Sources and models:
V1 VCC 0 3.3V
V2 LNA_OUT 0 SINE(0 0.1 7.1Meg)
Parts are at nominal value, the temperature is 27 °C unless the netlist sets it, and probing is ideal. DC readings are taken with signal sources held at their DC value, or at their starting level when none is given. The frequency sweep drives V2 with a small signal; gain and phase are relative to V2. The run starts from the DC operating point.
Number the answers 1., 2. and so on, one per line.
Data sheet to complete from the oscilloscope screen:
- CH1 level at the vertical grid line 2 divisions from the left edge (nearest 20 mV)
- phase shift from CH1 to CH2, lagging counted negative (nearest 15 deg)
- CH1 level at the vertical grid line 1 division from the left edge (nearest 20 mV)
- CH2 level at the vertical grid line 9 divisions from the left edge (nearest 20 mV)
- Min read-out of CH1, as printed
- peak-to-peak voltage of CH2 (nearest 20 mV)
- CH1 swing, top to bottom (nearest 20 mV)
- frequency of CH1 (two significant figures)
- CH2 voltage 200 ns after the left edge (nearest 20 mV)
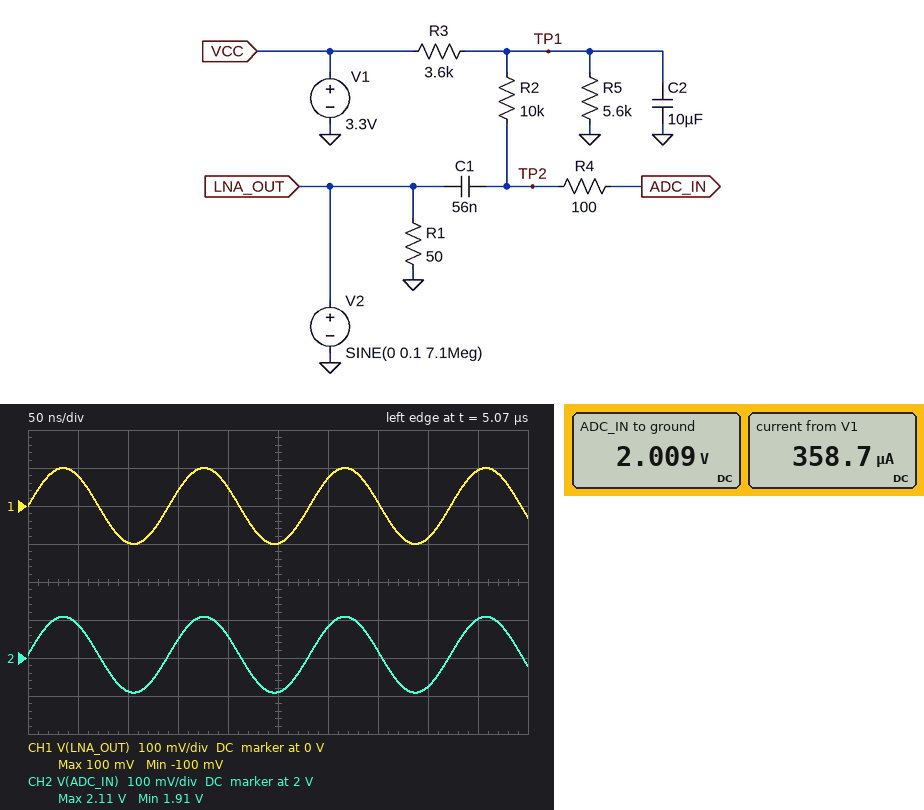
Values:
1. -100 mV
2. 0 deg
3. 80 mV
4. 2.10 V
5. -100 mV
6. 200 mV
7. 200 mV
8. 7.1 MHz
9. 2.06 V
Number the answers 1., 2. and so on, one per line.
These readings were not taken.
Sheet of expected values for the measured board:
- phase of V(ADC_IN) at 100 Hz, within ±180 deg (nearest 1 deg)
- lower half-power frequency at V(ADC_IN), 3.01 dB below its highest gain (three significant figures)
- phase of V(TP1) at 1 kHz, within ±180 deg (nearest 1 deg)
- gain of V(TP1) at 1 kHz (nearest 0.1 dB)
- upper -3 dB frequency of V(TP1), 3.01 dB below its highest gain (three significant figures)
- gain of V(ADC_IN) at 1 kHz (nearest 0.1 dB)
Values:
1. 70 deg
2. 286 Hz
3. -74 deg
4. -56.3 dB
5. 300 Hz
6. -0.3 dB
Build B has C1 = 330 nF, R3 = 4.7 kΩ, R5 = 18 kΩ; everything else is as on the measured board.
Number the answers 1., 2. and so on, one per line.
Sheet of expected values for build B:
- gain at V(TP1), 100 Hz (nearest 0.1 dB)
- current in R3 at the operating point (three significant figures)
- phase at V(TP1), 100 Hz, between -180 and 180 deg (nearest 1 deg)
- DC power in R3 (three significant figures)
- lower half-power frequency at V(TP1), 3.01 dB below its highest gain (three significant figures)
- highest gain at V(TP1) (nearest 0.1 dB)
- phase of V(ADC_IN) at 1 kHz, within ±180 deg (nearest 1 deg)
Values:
1. -36.9 dB
2. 145 µA
3. -61 deg
4. 99.3 µW
5. 3.57 Hz
6. -30.6 dB
7. 3 deg
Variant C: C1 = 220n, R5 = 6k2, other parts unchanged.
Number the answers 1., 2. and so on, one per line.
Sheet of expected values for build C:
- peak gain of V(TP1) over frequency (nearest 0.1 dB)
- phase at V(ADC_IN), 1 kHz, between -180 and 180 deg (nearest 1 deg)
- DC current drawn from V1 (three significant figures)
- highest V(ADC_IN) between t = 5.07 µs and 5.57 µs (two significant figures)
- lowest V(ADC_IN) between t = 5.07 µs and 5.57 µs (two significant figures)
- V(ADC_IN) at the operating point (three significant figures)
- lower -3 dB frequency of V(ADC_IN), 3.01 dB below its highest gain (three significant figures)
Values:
1. -34.1 dB
2. 4 deg
3. 337 µA
4. 2.2 V
5. 2.0 V
6. 2.09 V
7. 73.7 Hz
